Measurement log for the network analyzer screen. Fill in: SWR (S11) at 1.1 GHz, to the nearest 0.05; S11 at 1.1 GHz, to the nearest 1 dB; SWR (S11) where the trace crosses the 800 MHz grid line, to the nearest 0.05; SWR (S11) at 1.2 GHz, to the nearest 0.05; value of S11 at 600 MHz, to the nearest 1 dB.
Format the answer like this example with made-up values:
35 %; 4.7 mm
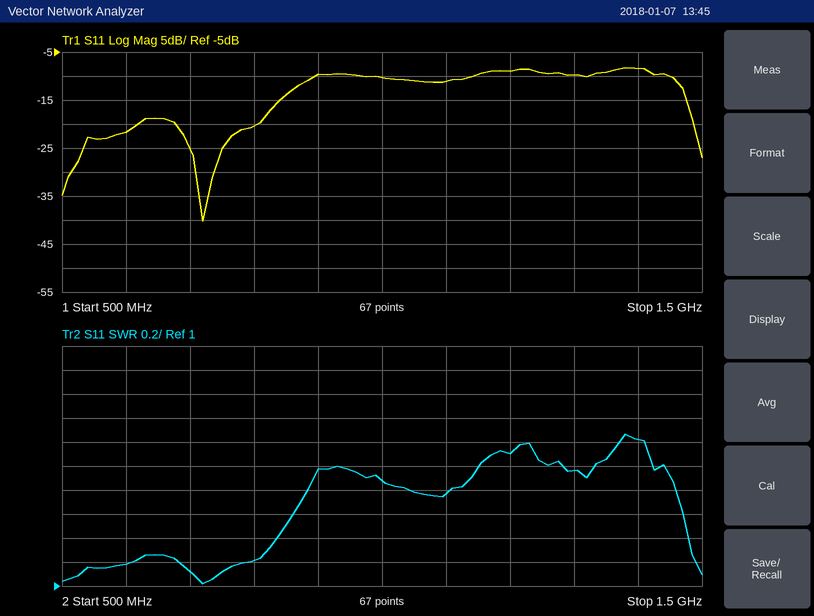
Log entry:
1.75; -11 dB; 1.20; 2.10; -22 dB
